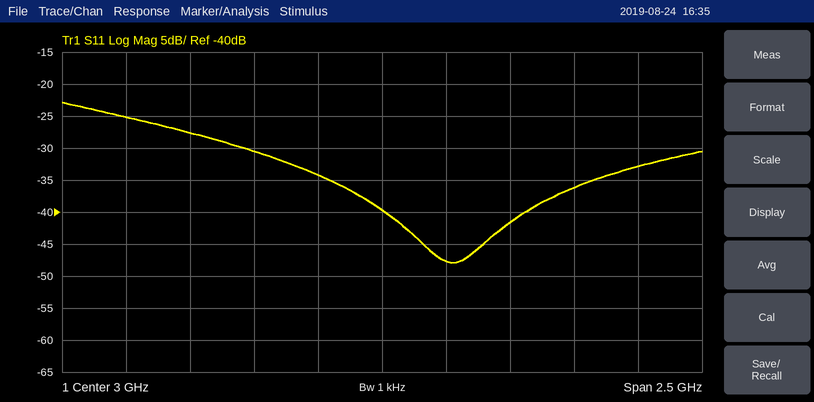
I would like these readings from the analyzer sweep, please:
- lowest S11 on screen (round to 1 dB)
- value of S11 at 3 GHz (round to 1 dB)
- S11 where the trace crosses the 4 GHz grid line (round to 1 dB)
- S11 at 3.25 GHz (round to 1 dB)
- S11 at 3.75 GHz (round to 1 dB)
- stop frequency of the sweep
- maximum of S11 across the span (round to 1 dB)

-48 dB
-40 dB
-33 dB
-48 dB
-36 dB
4.25 GHz
-23 dB
